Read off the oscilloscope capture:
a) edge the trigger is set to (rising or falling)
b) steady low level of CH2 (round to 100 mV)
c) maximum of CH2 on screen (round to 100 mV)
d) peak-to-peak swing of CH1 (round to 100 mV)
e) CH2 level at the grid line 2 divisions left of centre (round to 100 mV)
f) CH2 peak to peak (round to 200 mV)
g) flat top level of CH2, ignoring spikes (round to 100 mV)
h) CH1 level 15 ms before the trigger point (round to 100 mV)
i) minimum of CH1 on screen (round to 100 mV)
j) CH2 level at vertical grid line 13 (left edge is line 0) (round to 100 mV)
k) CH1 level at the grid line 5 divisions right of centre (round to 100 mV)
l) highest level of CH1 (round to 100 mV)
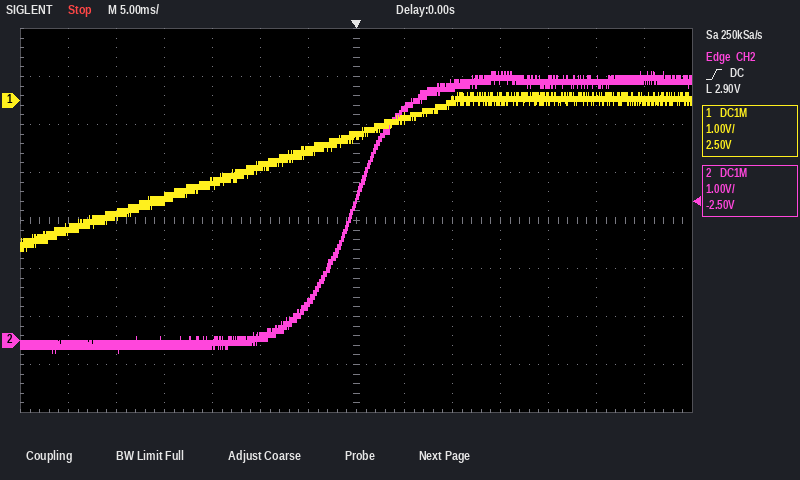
rising
-100 mV
5.6 V
3.3 V
100 mV
5.8 V
5.4 V
-1.7 V
-3.1 V
5.4 V
100 mV
200 mV
